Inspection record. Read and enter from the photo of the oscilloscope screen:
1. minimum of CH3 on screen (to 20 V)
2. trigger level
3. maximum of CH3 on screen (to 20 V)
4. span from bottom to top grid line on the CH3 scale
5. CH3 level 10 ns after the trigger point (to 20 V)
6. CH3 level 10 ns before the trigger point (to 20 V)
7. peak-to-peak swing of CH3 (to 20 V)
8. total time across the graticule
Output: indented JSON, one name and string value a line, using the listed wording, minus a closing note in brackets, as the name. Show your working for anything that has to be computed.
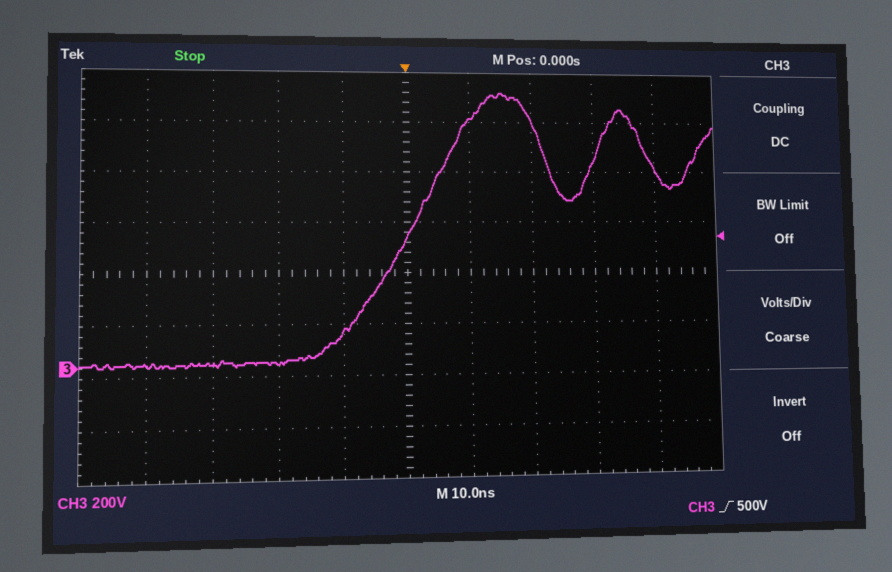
{
  "minimum of CH3 on screen": "0 V",
  "trigger level": "500 V",
  "maximum of CH3 on screen": "1.08 kV",
  "span from bottom to top grid line on the CH3 scale": "1.6 kV",
  "CH3 level 10 ns after the trigger point": "960 V",
  "CH3 level 10 ns before the trigger point": "120 V",
  "peak-to-peak swing of CH3": "1.08 kV − (0 V) = 1.08 kV",
  "total time across the graticule": "100 ns"
}
